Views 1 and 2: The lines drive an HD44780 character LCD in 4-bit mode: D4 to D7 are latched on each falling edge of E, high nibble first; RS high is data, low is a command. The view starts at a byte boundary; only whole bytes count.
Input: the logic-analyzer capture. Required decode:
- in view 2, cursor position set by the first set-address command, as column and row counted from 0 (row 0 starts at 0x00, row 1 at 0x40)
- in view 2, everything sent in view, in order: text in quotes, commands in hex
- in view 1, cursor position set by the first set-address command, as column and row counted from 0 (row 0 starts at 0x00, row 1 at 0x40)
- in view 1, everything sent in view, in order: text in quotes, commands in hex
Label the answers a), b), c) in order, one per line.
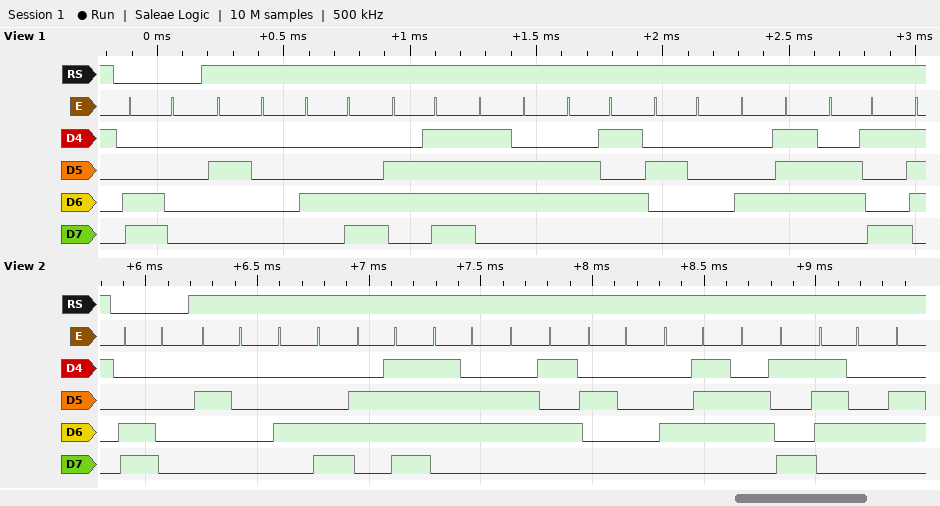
a) column 0, row 1
b) 0xC0 " Love Git"
c) column 0, row 1
d) 0xC0 " Love Gi"
